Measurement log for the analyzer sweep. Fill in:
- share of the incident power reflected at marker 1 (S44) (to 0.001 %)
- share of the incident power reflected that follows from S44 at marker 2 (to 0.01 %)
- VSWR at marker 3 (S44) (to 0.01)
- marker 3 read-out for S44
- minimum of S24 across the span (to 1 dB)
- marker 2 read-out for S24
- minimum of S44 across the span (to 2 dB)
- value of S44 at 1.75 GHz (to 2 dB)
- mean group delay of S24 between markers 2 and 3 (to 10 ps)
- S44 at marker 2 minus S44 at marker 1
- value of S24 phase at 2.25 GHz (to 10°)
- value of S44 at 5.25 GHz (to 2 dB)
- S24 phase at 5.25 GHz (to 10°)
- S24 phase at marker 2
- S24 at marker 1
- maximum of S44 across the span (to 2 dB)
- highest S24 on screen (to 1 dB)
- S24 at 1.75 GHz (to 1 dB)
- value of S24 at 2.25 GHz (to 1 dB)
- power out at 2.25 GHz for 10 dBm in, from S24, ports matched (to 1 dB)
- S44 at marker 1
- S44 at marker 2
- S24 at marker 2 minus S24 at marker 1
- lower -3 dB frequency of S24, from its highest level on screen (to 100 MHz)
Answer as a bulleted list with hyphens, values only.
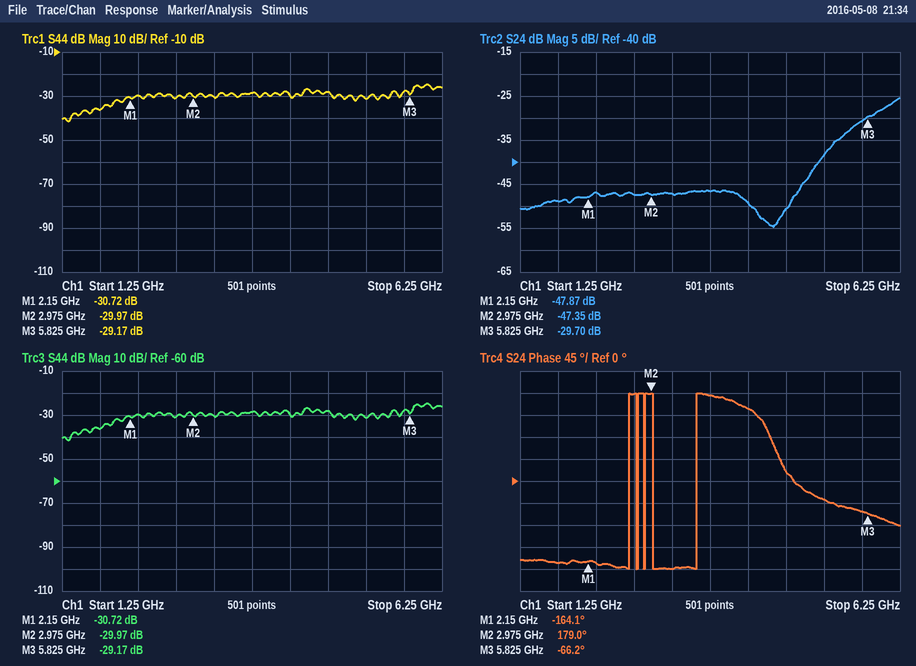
- 0.085 %
- 0.10 %
- 1.07
- -29.17 dB
- -55 dB
- -47.35 dB
- -42 dB
- -36 dB
- 240 ps
- 0.75 dB
- -170°
- -32 dB
- -40°
- 179.0°
- -47.87 dB
- -24 dB
- -25 dB
- -49 dB
- -47 dB
- -37 dBm
- -30.72 dB
- -29.97 dB
- 0.52 dB
- 6.0 GHz
